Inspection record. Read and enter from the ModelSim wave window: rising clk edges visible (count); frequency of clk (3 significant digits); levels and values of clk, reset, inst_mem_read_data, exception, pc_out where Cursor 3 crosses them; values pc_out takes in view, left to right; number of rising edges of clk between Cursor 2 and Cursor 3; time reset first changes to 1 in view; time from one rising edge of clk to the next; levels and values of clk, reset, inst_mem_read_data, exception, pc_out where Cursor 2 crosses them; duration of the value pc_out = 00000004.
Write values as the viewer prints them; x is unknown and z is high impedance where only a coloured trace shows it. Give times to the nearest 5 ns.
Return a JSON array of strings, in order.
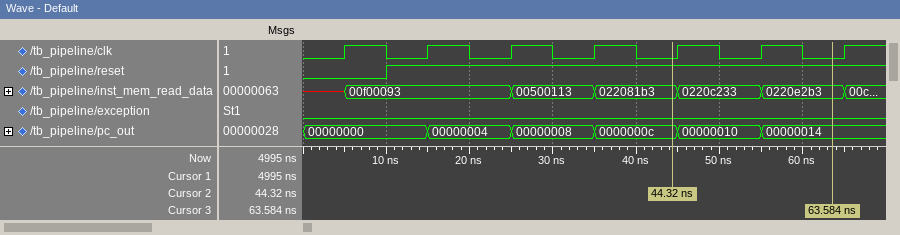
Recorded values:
["7", "100 MHz", "clk=0, reset=1, inst_mem_read_data=0220e2b3, exception=0, pc_out=00000014", "00000000, 00000004, 00000008, 0000000c, 00000010, 00000014", "2", "10 ns", "10 ns", "clk=0, reset=1, inst_mem_read_data=022081b3, exception=0, pc_out=0000000c", "10 ns"]
